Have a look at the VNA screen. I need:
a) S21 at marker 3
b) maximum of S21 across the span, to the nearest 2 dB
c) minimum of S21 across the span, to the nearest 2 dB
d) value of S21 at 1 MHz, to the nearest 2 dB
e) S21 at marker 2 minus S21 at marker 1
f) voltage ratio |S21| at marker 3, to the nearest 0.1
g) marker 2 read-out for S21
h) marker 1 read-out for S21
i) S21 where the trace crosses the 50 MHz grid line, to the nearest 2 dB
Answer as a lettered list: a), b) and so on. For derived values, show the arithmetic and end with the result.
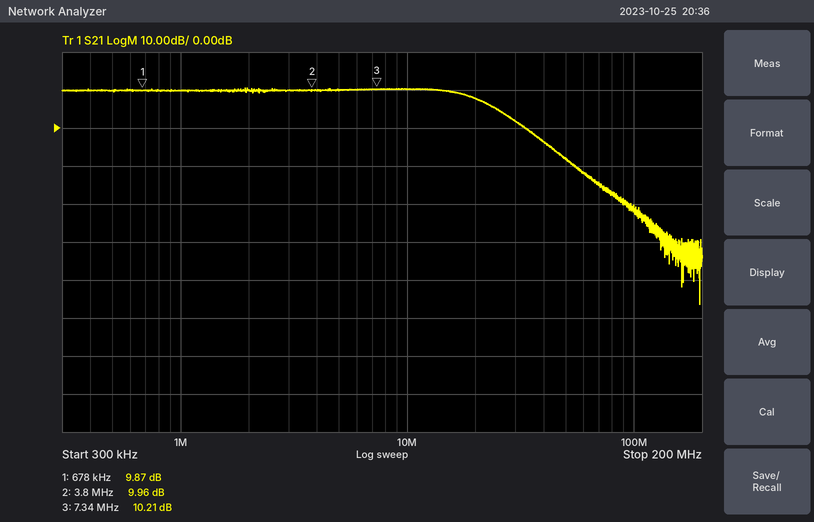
a) 10.21 dB
b) 10 dB
c) -46 dB
d) 10 dB
e) 9.96 − (9.87) = 0.09 dB
f) 10^(10.21/20) ≈ 3.2
g) 9.96 dB
h) 9.87 dB
i) -8 dB
